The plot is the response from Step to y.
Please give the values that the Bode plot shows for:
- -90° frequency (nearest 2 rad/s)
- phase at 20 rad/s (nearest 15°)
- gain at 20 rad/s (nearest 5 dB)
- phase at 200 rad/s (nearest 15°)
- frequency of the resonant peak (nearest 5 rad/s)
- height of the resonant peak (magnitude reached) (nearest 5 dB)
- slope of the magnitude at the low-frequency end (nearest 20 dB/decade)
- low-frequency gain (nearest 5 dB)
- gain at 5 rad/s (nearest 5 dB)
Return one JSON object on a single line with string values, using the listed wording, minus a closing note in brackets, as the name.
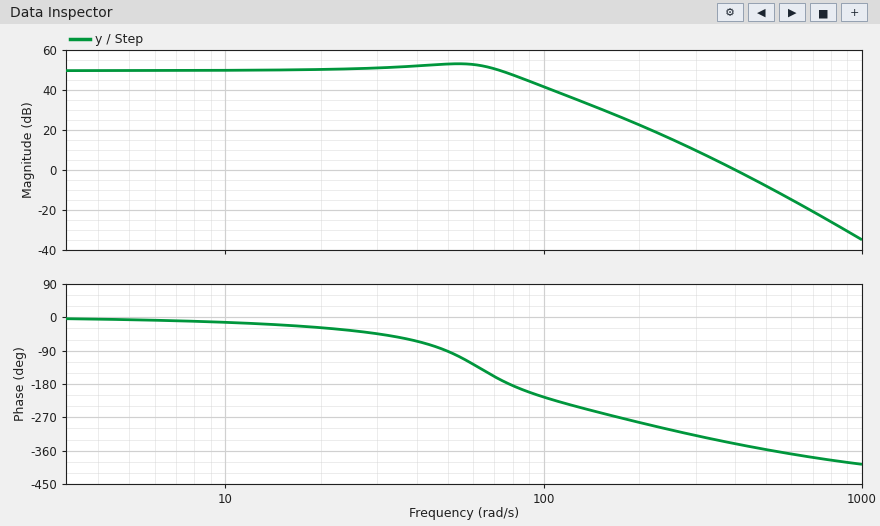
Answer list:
{"-90° frequency": "50 rad/s", "phase at 20 rad/s": "-30°", "gain at 20 rad/s": "50 dB", "phase at 200 rad/s": "-285°", "frequency of the resonant peak": "55 rad/s", "height of the resonant peak (magnitude reached)": "55 dB", "slope of the magnitude at the low-frequency end": "0 dB/decade", "low-frequency gain": "50 dB", "gain at 5 rad/s": "50 dB"}
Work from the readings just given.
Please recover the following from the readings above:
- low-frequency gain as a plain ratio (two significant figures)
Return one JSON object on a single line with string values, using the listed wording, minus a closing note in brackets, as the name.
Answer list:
{"low-frequency gain as a plain ratio": "320"}
